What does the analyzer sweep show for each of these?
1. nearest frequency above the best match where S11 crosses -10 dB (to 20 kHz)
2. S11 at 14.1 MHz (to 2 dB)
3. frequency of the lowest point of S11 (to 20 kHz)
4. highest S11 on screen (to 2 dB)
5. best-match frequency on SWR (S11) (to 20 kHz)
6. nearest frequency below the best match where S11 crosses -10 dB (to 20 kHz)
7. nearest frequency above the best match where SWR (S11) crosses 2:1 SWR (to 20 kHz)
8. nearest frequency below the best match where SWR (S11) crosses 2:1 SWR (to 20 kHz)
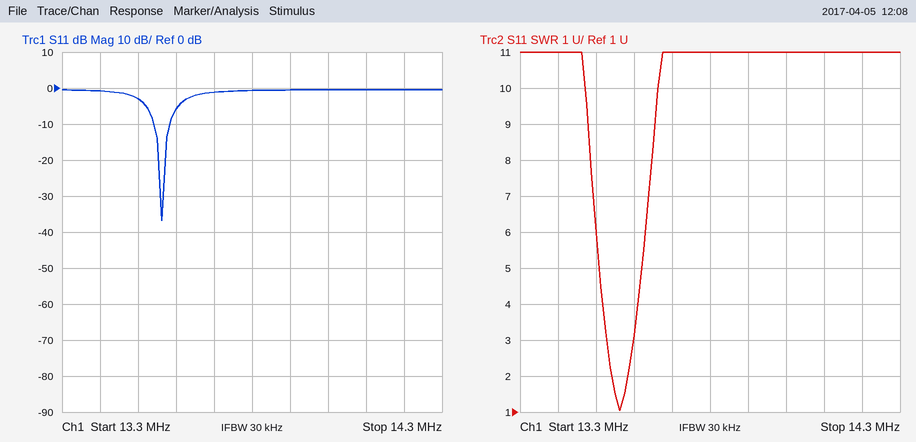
13.58 MHz
0 dB
13.56 MHz
0 dB
13.56 MHz
13.54 MHz
13.58 MHz
13.54 MHz
